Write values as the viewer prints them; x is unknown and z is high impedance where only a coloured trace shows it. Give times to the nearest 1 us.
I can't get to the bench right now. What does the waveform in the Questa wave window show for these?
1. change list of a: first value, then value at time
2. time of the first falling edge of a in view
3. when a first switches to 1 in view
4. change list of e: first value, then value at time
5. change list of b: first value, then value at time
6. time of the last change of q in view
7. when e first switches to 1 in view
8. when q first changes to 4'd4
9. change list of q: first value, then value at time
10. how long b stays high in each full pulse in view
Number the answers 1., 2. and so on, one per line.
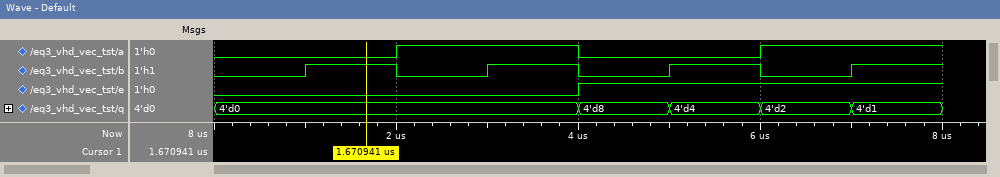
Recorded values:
1. 0, 1 at 2 us, 0 at 4 us, 1 at 6 us
2. 4 us
3. 2 us
4. 0, 1 at 4 us
5. 0, 1 at 1 us, 0 at 2 us, 1 at 3 us, 0 at 4 us, 1 at 5 us, 0 at 6 us, 1 at 7 us
6. 7 us
7. 4 us
8. 5 us
9. 4'd0, 4'd8 at 4 us, 4'd4 at 5 us, 4'd2 at 6 us, 4'd1 at 7 us
10. 1 us, 1 us, 1 us
